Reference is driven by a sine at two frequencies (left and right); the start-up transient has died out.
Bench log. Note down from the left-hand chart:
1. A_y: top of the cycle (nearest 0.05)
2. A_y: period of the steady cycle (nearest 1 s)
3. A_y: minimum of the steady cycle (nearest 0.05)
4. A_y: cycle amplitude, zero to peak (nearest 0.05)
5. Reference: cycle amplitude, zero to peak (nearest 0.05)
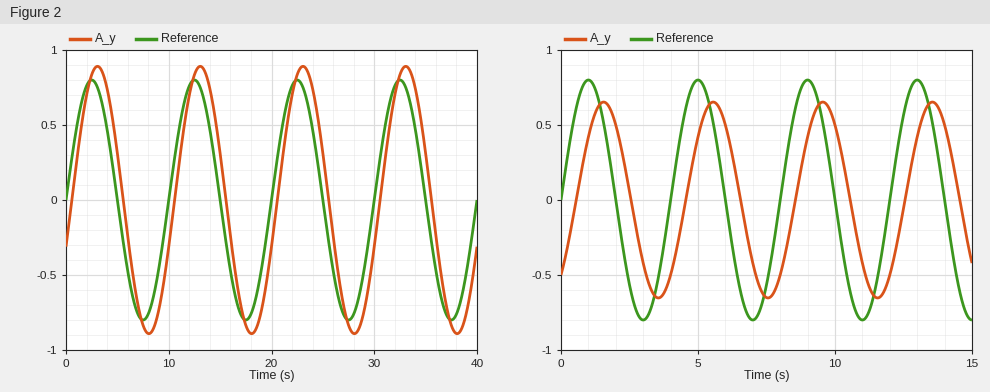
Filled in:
0.90
10 s
-0.90
0.90
0.80
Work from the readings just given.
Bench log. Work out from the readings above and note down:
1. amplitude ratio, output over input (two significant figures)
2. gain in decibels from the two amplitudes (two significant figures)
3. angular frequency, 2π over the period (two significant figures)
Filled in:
1.1
1.0 dB
0.63 rad/s
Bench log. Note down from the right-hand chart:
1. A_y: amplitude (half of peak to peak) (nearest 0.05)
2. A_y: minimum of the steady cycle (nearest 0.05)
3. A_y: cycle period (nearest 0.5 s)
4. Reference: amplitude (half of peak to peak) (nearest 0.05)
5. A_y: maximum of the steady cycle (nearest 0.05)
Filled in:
0.65
-0.65
4.0 s
0.80
0.65
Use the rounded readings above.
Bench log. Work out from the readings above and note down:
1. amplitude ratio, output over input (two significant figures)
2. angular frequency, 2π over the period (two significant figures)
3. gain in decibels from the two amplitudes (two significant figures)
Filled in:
0.81
1.6 rad/s
-1.8 dB
